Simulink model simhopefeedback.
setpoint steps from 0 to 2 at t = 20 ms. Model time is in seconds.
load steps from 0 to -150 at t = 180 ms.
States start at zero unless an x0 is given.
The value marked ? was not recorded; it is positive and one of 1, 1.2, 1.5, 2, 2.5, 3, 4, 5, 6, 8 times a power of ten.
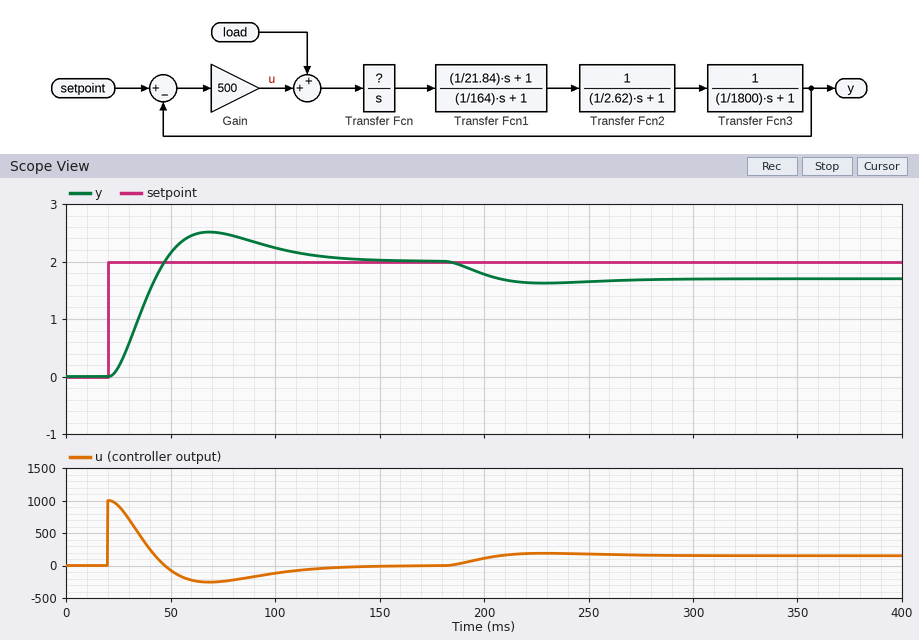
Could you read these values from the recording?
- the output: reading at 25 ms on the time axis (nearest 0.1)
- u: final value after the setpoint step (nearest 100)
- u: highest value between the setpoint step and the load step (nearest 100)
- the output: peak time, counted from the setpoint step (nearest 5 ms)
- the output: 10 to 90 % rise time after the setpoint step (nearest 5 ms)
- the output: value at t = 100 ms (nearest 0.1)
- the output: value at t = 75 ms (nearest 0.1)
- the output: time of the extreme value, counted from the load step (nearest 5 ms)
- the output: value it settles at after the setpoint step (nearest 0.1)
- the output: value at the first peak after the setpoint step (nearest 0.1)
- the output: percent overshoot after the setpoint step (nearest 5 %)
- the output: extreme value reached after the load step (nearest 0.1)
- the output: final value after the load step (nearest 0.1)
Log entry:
0.2
0
1000
50 ms
20 ms
2.2
2.5
50 ms
2.0
2.5
25 %
1.6
1.7
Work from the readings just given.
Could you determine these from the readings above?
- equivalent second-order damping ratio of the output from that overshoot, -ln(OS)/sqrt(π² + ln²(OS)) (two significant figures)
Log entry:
0.40
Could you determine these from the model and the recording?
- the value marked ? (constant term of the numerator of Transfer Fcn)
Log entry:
1
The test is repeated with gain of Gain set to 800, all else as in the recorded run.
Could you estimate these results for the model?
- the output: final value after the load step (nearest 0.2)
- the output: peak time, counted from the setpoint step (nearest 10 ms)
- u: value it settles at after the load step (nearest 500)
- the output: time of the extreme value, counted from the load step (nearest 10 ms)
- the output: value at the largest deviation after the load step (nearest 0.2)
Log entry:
1.8
30 ms
0
30 ms
1.8
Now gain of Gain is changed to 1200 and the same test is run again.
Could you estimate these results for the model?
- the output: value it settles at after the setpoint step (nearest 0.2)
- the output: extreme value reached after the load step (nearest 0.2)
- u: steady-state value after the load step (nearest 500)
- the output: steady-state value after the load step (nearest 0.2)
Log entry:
2.0
1.8
0
1.8
